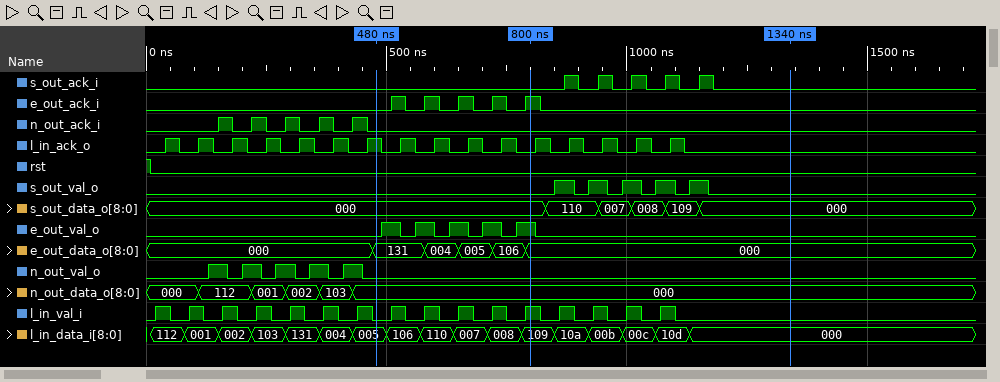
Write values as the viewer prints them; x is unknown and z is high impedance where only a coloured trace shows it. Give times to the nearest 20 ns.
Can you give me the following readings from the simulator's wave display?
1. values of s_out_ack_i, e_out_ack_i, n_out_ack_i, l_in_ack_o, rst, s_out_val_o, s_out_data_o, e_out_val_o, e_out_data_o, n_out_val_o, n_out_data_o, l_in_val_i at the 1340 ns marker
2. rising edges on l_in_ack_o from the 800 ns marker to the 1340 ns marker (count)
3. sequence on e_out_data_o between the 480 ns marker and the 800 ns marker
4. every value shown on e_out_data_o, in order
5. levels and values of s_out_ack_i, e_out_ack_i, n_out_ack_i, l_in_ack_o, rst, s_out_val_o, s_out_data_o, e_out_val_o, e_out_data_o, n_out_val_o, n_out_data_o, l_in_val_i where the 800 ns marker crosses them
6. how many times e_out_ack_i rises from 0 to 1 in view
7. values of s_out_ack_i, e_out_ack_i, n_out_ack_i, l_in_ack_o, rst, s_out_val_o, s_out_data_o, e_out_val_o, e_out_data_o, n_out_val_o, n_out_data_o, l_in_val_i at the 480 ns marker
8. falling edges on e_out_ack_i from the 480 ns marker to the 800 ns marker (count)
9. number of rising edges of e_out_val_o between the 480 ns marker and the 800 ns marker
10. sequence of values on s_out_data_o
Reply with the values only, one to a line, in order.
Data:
s_out_ack_i=0, e_out_ack_i=0, n_out_ack_i=0, l_in_ack_o=0, rst=0, s_out_val_o=0, s_out_data_o=000, e_out_val_o=0, e_out_data_o=000, n_out_val_o=0, n_out_data_o=000, l_in_val_i=0
5
131, 004, 005, 106, 000
000, 131, 004, 005, 106, 000
s_out_ack_i=0, e_out_ack_i=1, n_out_ack_i=0, l_in_ack_o=0, rst=0, s_out_val_o=0, s_out_data_o=000, e_out_val_o=1, e_out_data_o=000, n_out_val_o=0, n_out_data_o=000, l_in_val_i=1
5
s_out_ack_i=0, e_out_ack_i=0, n_out_ack_i=0, l_in_ack_o=1, rst=0, s_out_val_o=0, s_out_data_o=000, e_out_val_o=0, e_out_data_o=131, n_out_val_o=0, n_out_data_o=000, l_in_val_i=0
4
5
000, 110, 007, 008, 109, 000
